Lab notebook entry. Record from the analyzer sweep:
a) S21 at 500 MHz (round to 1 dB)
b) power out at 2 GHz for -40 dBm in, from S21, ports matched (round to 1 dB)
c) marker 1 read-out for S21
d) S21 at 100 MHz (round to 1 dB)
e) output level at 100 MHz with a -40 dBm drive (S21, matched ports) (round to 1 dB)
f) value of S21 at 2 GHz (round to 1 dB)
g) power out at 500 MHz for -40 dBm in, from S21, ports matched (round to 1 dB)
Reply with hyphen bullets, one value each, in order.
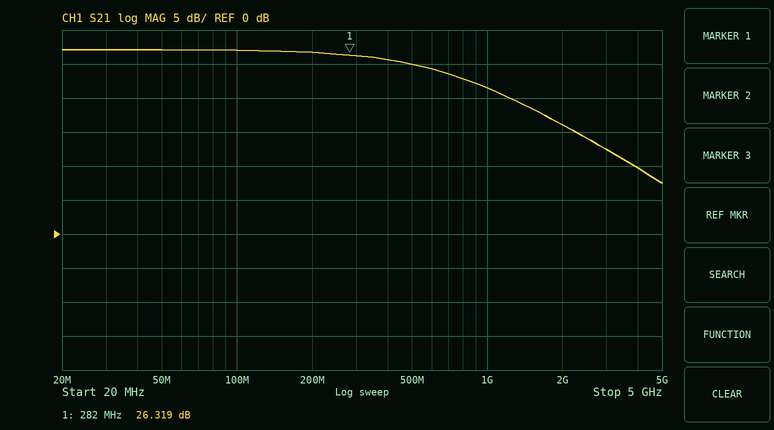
- 25 dB
- -24 dBm
- 26.319 dB
- 27 dB
- -13 dBm
- 16 dB
- -15 dBm
